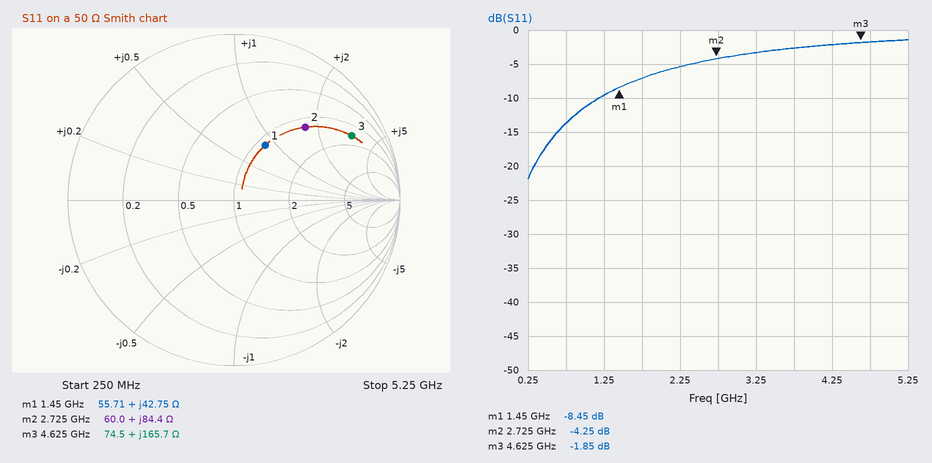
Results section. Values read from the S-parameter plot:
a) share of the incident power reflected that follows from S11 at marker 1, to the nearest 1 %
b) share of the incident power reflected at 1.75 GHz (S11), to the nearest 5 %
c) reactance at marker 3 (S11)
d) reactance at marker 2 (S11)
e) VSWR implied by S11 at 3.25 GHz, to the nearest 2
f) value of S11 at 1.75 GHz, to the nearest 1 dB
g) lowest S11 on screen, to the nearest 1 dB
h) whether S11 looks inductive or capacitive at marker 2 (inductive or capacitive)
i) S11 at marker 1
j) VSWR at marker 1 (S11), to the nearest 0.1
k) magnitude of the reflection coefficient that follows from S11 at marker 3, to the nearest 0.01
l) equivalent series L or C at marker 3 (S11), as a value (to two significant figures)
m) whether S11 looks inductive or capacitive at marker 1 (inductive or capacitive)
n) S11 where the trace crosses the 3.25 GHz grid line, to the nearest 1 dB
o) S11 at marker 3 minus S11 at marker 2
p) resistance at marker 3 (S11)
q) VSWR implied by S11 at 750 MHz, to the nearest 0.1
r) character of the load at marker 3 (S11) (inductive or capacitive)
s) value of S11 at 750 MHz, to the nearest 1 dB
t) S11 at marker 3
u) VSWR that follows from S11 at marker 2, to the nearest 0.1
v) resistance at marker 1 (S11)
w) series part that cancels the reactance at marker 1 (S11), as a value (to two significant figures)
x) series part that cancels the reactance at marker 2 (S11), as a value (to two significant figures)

14 %
20 %
+165.7 Ω
+84.4 Ω
6
-7 dB
-22 dB
inductive
-8.45 dB
2.2
0.81
5.7 nH
inductive
-3 dB
2.40 dB
74.5 Ω
1.5
inductive
-14 dB
-1.85 dB
4.2
55.71 Ω
2.6 pF
690 fF
